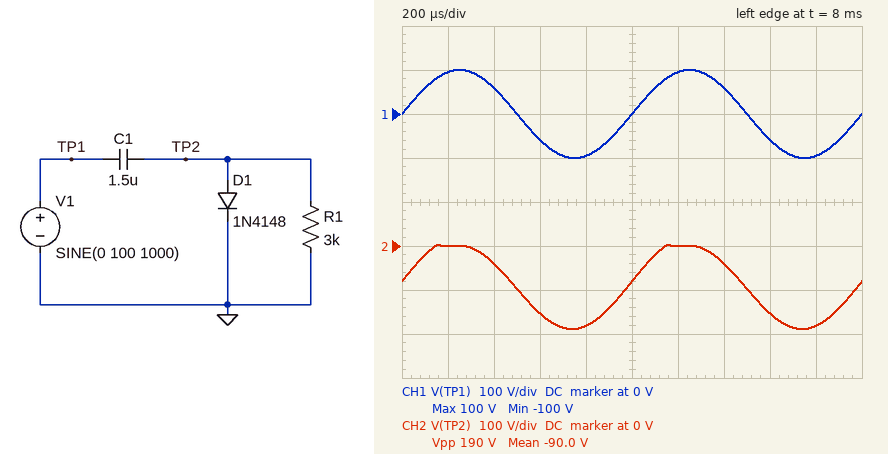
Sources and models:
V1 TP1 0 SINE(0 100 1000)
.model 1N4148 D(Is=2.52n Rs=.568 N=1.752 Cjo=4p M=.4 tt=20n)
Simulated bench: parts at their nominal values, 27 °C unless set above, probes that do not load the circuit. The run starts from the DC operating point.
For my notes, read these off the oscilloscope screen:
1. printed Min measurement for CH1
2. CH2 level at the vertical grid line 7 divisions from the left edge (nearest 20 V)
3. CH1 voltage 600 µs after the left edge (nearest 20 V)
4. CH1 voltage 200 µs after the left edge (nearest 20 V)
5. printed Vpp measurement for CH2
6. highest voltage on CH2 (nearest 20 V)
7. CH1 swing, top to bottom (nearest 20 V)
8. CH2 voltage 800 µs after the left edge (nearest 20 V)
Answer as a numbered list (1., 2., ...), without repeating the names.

1. -100 V
2. -40 V
3. -60 V
4. 100 V
5. 190 V
6. 0 V
7. 200 V
8. -180 V
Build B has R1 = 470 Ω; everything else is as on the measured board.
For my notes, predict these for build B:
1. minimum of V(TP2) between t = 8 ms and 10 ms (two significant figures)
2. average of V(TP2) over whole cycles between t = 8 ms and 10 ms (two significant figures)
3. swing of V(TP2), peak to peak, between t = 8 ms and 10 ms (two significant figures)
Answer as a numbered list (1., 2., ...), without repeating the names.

1. -150 V
2. -62 V
3. 150 V
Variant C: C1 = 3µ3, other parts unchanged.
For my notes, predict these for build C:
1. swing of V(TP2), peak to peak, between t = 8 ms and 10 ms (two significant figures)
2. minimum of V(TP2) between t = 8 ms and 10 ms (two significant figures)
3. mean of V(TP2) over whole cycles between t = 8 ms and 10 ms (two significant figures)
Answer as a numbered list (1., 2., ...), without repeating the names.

1. 200 V
2. -190 V
3. -95 V
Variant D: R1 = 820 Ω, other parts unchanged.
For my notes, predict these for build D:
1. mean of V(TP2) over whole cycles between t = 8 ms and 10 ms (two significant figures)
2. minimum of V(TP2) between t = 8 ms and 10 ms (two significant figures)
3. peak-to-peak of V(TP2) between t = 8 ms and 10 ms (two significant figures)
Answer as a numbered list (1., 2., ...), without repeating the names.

1. -74 V
2. -170 V
3. 170 V
